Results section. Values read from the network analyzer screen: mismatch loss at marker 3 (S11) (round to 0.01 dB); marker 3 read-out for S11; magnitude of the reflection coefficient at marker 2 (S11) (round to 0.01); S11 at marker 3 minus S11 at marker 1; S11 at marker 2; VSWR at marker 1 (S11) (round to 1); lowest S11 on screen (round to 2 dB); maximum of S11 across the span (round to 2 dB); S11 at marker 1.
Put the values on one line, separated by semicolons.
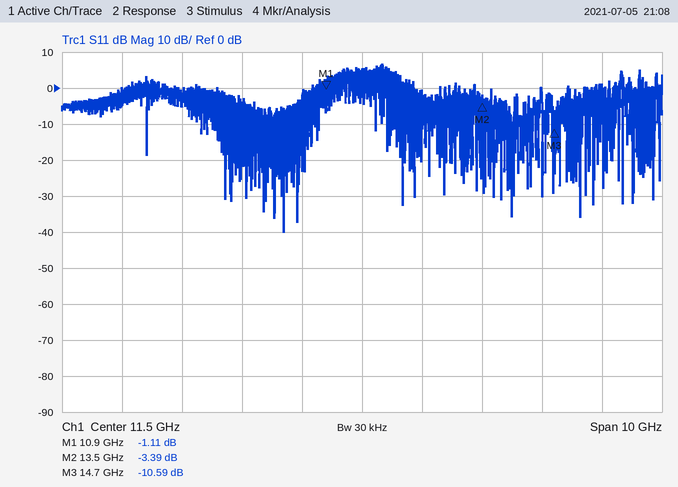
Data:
0.40 dB; -10.59 dB; 0.68; -9.48 dB; -3.39 dB; 16; -40 dB; 6 dB; -1.11 dB
